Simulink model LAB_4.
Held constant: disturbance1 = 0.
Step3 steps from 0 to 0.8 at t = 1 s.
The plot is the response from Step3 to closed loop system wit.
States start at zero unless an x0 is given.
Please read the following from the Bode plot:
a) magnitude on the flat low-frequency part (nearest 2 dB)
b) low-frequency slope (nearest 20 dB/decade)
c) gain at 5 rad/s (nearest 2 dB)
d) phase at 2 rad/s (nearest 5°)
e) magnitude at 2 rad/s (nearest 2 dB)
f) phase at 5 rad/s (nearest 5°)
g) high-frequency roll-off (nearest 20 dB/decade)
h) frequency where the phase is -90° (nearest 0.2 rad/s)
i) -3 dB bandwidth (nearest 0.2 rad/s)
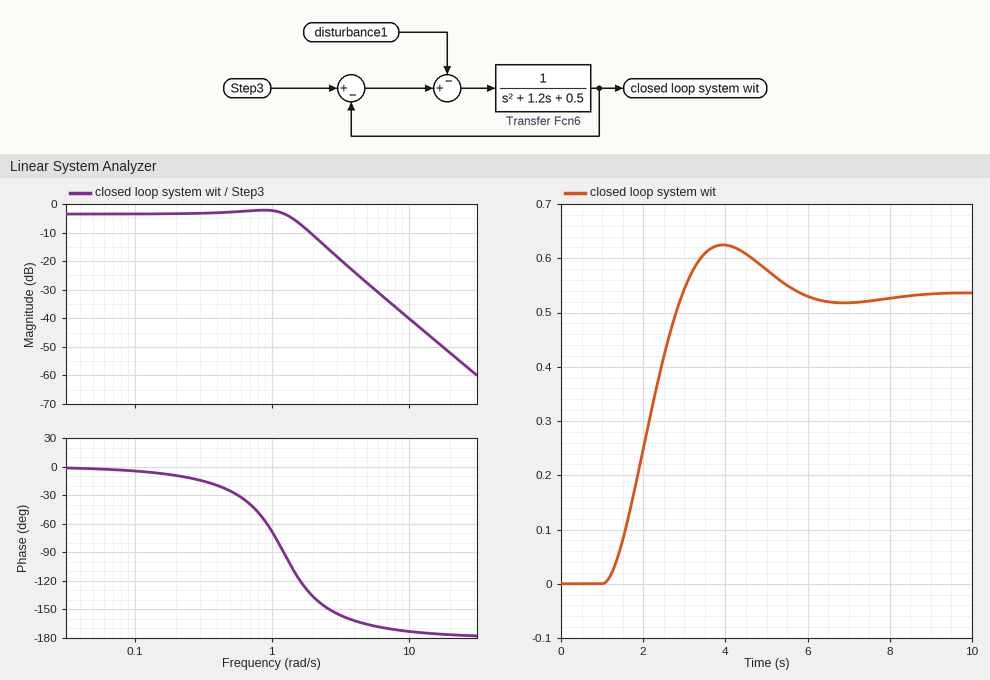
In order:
-4 dB
0 dB/decade
-28 dB
-135°
-10 dB
-165°
-40 dB/decade
1.2 rad/s
1.6 rad/s
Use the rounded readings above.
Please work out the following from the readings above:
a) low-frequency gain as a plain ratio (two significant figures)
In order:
0.63
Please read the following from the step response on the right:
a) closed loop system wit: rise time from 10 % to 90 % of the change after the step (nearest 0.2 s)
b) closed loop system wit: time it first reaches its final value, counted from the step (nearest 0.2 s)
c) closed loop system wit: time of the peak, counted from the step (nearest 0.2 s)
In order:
1.4 s
2.0 s
3.0 s
